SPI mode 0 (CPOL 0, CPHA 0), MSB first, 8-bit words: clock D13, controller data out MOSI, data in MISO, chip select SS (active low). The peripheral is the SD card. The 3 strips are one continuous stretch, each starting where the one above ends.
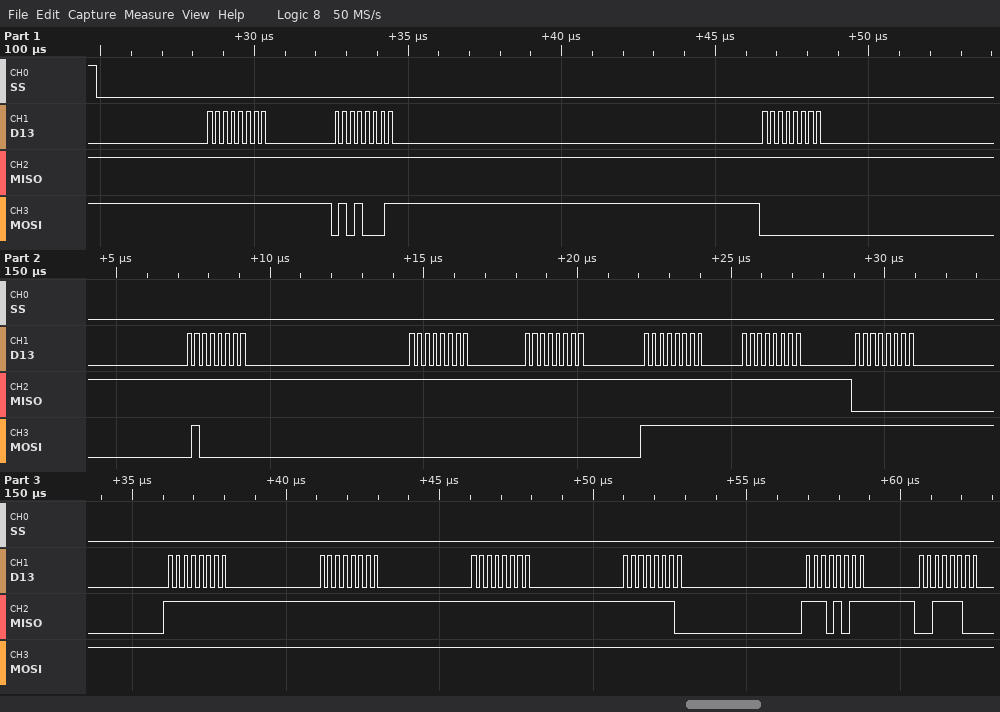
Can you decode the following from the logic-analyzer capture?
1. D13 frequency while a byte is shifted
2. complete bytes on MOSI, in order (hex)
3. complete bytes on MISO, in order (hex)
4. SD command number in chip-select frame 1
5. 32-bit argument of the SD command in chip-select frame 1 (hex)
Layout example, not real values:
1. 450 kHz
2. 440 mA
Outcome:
1. 4 MHz
2. FF 51 00 40 00 00 FF FF FF FF FF FF FF FF FF
3. FF FF FF FF FF FF FF FF 00 FF FF FF FE EB 3C
4. CMD17
5. 0x00400000
